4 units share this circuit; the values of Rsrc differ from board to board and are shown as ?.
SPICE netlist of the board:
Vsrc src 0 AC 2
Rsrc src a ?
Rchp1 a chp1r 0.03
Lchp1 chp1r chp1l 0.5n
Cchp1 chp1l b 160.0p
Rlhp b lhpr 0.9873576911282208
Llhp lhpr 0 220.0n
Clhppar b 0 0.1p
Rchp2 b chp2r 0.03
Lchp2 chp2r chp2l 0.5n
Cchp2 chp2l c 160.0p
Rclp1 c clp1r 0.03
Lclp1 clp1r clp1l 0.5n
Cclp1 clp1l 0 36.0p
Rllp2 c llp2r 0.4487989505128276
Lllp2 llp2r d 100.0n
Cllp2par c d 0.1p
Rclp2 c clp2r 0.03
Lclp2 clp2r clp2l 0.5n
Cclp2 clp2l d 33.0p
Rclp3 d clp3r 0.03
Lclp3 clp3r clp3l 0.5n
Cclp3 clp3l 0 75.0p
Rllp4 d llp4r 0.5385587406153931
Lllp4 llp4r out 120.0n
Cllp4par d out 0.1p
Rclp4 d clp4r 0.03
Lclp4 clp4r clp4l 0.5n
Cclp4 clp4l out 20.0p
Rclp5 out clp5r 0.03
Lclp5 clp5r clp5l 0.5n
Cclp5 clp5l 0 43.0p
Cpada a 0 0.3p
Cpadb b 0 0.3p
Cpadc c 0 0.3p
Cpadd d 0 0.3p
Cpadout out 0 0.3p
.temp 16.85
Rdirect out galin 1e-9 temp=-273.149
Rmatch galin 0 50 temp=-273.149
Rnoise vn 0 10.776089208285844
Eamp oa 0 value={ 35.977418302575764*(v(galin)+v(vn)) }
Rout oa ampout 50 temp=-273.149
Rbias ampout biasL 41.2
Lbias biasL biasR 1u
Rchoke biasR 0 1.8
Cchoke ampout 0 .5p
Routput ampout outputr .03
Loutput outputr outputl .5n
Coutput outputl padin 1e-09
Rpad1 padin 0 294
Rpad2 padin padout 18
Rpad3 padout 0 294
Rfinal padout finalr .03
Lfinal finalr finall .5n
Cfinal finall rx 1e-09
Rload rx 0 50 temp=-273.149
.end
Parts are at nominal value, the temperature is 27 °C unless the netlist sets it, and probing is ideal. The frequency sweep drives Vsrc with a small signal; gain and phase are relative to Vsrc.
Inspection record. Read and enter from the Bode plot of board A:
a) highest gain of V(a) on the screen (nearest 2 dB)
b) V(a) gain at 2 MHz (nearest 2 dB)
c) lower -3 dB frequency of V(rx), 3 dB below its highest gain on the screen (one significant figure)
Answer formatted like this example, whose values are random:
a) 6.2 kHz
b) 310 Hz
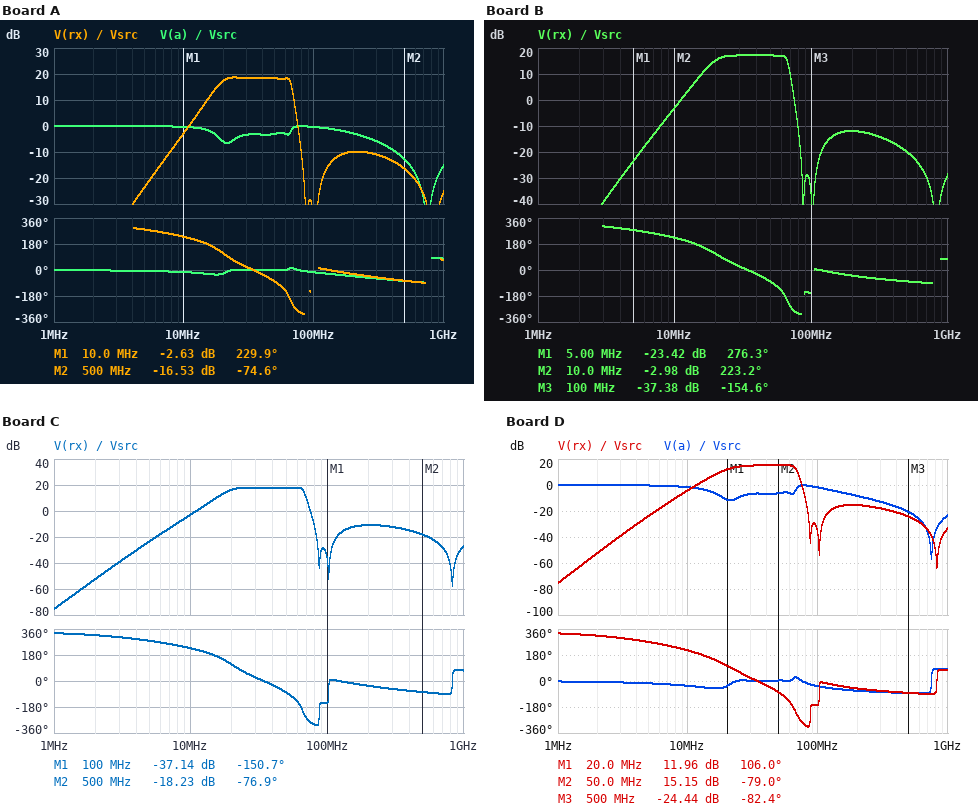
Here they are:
a) 0 dB
b) 0 dB
c) 20 MHz
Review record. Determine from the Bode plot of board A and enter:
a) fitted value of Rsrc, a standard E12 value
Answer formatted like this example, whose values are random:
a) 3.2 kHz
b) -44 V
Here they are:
a) 22 Ω
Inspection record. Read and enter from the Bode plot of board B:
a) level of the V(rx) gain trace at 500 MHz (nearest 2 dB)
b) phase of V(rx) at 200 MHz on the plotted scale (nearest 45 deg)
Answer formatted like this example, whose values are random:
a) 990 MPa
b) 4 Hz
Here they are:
a) -20 dB
b) -45 deg
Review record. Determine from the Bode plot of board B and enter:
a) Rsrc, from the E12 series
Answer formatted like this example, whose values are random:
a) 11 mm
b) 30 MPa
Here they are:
a) 33 Ω
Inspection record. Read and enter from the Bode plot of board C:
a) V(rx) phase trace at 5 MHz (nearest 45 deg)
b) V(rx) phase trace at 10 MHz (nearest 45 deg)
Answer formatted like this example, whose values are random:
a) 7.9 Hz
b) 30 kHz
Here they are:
a) 270 deg
b) 225 deg
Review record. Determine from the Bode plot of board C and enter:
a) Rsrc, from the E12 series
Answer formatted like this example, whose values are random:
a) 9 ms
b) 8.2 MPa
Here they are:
a) 27 Ω
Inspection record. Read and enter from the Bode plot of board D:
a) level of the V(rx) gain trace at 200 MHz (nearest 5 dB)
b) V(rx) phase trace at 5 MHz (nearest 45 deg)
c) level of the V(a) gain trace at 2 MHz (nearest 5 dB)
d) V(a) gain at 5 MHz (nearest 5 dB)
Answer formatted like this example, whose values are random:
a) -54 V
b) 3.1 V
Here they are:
a) -15 dB
b) 270 deg
c) 0 dB
d) 0 dB
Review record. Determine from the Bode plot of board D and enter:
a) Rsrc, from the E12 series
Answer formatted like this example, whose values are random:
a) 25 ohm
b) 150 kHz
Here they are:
a) 56 Ω
